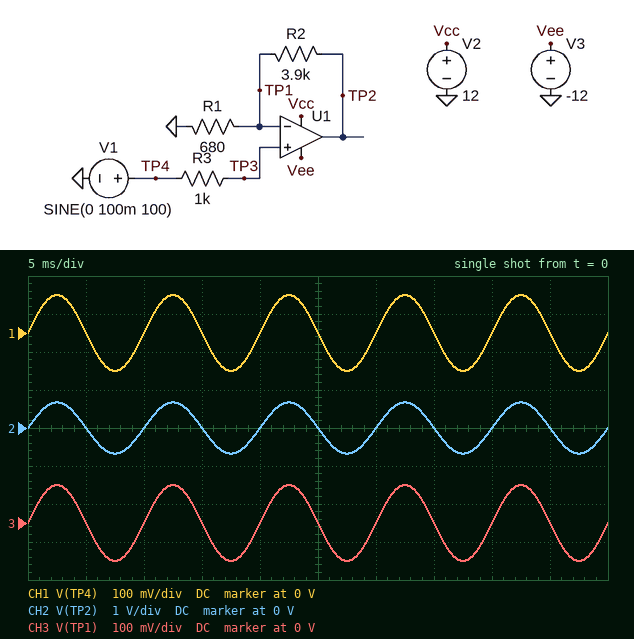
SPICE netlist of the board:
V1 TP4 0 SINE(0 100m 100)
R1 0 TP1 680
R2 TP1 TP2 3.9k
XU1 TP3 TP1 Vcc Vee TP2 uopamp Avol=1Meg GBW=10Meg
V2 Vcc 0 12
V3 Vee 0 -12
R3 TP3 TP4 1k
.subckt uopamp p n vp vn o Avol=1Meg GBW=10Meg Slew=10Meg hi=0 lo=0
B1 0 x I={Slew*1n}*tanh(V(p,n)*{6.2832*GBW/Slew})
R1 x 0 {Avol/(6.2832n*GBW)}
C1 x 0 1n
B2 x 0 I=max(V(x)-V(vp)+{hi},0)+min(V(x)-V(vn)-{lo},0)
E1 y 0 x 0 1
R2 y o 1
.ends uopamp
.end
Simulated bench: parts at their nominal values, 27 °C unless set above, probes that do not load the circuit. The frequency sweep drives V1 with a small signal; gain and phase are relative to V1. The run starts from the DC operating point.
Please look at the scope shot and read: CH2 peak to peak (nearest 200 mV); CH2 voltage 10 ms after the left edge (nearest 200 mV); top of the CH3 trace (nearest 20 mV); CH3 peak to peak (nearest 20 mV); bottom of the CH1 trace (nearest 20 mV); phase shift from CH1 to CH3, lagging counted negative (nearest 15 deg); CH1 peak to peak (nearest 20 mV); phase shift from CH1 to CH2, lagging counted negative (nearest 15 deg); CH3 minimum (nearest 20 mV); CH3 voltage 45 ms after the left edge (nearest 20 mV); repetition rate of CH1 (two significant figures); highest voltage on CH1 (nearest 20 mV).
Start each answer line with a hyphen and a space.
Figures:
- 1.4 V
- 0 V
- 100 mV
- 200 mV
- -100 mV
- 0 deg
- 200 mV
- 0 deg
- -100 mV
- 0 V
- 100 Hz
- 100 mV
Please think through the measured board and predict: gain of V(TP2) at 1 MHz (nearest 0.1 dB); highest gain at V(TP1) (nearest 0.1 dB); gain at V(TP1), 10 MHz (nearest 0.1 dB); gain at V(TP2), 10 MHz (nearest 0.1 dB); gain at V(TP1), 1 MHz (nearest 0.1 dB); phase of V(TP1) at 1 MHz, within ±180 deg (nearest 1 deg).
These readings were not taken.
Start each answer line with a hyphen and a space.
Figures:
- 14.9 dB
- 0 dB
- -16.7 dB
- -0.1 dB
- -1.6 dB
- -34 deg
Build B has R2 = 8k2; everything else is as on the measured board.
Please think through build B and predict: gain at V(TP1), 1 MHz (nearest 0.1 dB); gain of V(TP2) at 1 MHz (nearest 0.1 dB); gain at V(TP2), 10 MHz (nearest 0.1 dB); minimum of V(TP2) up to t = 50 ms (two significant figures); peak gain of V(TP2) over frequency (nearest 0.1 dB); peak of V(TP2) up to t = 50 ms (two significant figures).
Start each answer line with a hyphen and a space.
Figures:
- -4.3 dB
- 18.0 dB
- 0 dB
- -1.3 V
- 22.3 dB
- 1.3 V
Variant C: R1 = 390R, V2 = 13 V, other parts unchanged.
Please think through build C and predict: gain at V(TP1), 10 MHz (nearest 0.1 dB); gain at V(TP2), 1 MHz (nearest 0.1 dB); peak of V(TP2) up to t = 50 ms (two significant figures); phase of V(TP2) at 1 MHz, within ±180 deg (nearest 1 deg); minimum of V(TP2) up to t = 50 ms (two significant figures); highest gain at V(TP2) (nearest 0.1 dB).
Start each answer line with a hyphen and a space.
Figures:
- -20.9 dB
- 17.4 dB
- 1.1 V
- -48 deg
- -1.1 V
- 20.8 dB
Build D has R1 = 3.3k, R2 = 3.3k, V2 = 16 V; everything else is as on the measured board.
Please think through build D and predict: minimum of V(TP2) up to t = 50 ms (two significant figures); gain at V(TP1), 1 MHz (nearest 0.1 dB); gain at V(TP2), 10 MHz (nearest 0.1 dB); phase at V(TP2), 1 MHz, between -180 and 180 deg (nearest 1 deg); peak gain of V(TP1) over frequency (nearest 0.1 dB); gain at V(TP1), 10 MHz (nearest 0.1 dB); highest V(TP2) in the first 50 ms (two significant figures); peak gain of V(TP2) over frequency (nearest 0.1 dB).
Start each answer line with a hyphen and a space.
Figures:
- -200 mV
- -0.2 dB
- -1.0 dB
- -11 deg
- 0 dB
- -7.0 dB
- 200 mV
- 6.0 dB
